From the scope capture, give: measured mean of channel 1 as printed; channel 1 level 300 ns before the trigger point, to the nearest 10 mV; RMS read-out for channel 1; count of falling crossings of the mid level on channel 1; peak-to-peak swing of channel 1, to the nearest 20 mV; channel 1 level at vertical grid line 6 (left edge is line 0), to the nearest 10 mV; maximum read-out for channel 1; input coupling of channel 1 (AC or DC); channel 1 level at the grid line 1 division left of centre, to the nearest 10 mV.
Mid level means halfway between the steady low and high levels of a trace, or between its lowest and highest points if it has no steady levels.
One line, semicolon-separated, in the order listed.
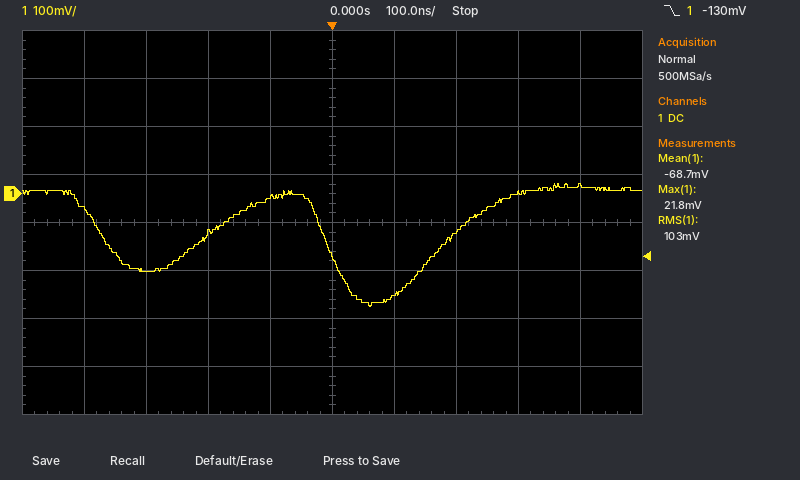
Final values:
-68.7 mV; -160 mV; 103 mV; 2; 260 mV; -210 mV; 21.8 mV; DC; -10 mV
